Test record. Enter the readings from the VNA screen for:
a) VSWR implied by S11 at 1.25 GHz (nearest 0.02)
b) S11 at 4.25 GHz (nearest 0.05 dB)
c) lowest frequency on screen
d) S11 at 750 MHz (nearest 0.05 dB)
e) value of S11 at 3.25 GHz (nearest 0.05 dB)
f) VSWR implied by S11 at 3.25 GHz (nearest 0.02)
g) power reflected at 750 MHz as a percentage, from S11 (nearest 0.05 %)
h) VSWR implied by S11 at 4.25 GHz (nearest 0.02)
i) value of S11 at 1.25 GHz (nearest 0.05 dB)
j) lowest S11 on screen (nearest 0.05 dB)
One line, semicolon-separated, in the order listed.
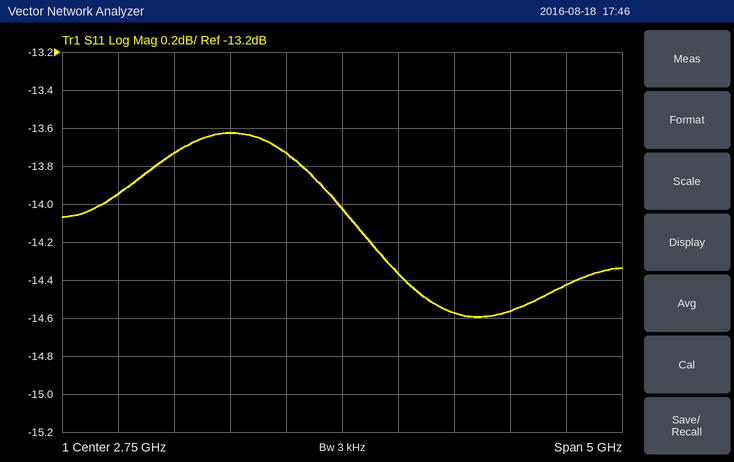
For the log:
1.52; -14.55 dB; 250 MHz; -13.95 dB; -14.35 dB; 1.48; 4.05 %; 1.46; -13.75 dB; -14.60 dB
